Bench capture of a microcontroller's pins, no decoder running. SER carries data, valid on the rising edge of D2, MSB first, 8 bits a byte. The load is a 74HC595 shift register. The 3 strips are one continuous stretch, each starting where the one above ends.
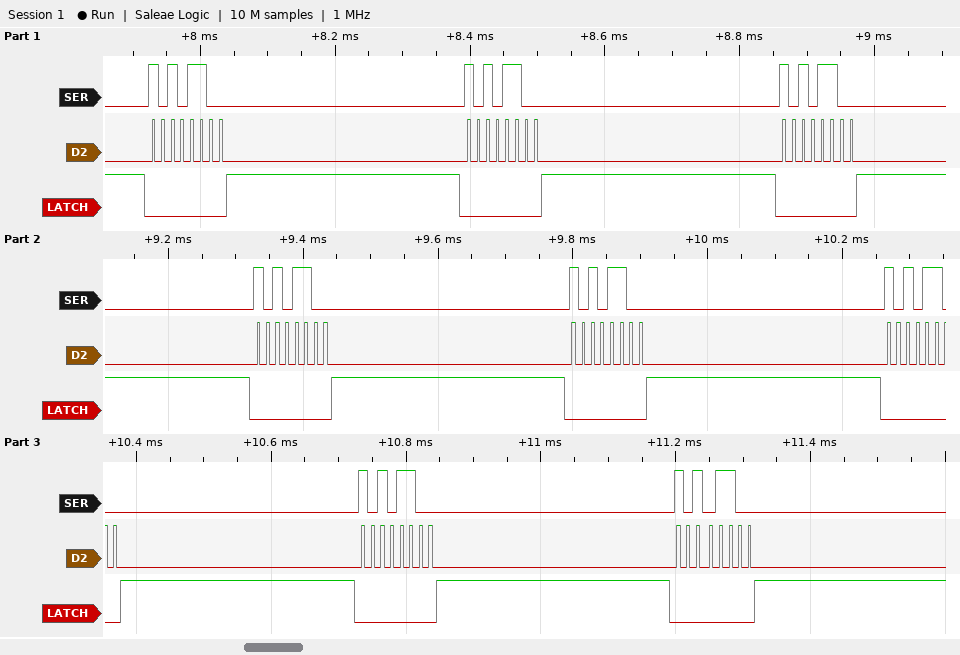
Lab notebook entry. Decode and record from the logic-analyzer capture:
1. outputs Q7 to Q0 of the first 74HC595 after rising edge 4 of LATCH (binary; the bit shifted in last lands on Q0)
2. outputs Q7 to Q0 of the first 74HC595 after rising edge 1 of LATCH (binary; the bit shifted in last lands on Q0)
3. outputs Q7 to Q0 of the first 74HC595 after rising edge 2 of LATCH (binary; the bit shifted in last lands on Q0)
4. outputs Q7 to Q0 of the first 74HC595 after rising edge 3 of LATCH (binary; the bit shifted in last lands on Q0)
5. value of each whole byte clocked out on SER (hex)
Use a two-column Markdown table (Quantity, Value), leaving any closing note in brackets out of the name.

| Quantity | Value |
|---|---|
| outputs Q7 to Q0 of the first 74HC595 after rising edge 4 of LATCH | 10101100 |
| outputs Q7 to Q0 of the first 74HC595 after rising edge 1 of LATCH | 10101100 |
| outputs Q7 to Q0 of the first 74HC595 after rising edge 2 of LATCH | 10101100 |
| outputs Q7 to Q0 of the first 74HC595 after rising edge 3 of LATCH | 10101100 |
| value of each whole byte clocked out on SER | AC AC AC AC AC AC AC AC |
